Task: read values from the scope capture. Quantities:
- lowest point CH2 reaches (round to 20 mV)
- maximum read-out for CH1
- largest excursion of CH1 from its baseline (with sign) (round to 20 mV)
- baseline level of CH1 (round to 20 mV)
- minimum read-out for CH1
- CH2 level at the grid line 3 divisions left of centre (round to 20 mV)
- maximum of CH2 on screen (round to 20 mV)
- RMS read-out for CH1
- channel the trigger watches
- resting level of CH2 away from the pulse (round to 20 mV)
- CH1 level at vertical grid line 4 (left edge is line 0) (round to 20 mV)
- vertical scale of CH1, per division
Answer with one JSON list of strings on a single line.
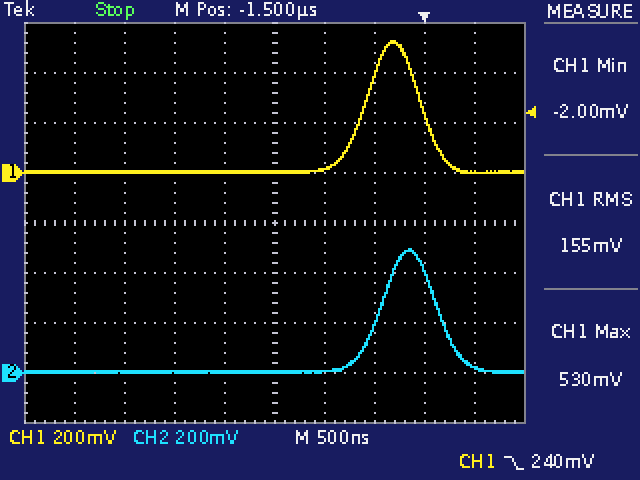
["0 mV", "530 mV", "+520 mV", "0 mV", "-2.00 mV", "0 mV", "500 mV", "155 mV", "CH1", "0 mV", "0 mV", "200 mV"]
